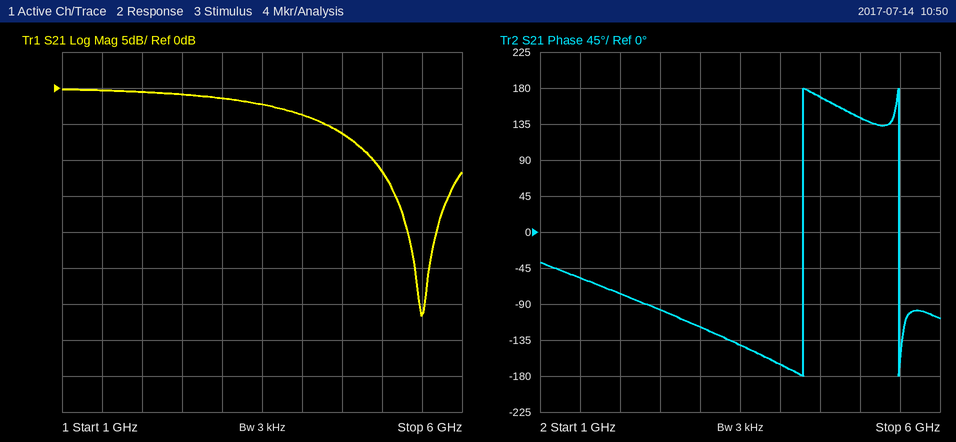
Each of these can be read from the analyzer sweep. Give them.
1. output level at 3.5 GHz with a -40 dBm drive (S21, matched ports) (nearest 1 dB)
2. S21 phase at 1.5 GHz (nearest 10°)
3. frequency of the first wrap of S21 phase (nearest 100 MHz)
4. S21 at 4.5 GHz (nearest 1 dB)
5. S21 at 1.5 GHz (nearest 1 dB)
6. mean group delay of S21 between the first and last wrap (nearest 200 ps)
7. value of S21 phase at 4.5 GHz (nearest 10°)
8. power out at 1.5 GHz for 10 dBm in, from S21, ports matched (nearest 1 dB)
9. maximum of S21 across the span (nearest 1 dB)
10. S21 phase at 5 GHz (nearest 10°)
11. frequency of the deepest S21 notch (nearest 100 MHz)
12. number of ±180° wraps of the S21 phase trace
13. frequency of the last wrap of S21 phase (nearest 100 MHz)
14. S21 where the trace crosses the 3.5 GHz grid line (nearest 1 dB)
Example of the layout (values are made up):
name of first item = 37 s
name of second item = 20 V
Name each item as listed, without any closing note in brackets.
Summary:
output level at 3.5 GHz with a -40 dBm drive (S21, matched ports) = -42 dBm
S21 phase at 1.5 GHz = -60°
frequency of the first wrap of S21 phase = 4.3 GHz
S21 at 4.5 GHz = -6 dB
S21 at 1.5 GHz = 0 dB
mean group delay of S21 between the first and last wrap = 800 ps
value of S21 phase at 4.5 GHz = 170°
power out at 1.5 GHz for 10 dBm in, from S21, ports matched = 10 dBm
maximum of S21 across the span = 0 dB
S21 phase at 5 GHz = 140°
frequency of the deepest S21 notch = 5.5 GHz
number of ±180° wraps of the S21 phase trace = 2
frequency of the last wrap of S21 phase = 5.5 GHz
S21 where the trace crosses the 3.5 GHz grid line = -2 dB
